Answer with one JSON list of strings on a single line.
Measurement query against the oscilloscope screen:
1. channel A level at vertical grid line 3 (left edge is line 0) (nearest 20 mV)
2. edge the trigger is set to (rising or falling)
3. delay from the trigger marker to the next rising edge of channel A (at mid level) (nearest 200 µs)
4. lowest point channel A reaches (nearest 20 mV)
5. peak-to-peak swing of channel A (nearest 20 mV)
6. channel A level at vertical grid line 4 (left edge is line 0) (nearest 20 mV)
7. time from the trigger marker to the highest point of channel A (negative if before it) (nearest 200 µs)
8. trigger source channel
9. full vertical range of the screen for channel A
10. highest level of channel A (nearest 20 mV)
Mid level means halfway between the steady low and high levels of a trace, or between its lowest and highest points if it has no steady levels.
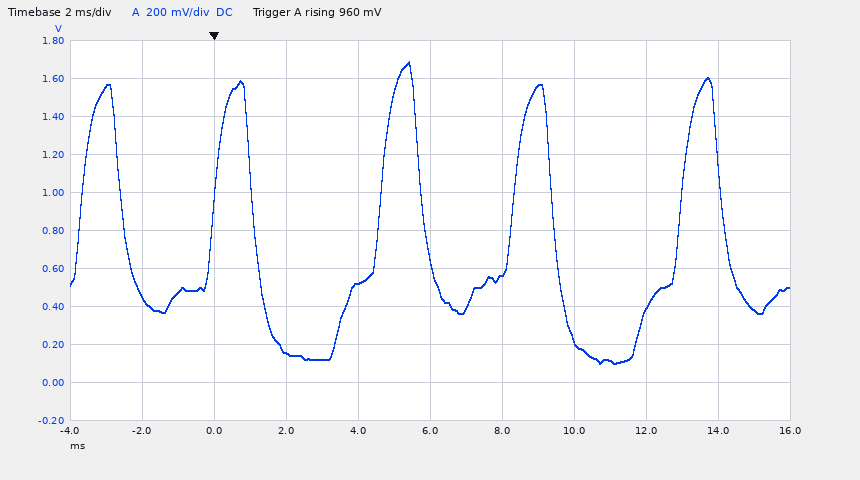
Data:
["160 mV", "rising", "4.6 ms", "100 mV", "1.58 V", "520 mV", "+5.4 ms", "channel A", "2 V", "1.68 V"]
